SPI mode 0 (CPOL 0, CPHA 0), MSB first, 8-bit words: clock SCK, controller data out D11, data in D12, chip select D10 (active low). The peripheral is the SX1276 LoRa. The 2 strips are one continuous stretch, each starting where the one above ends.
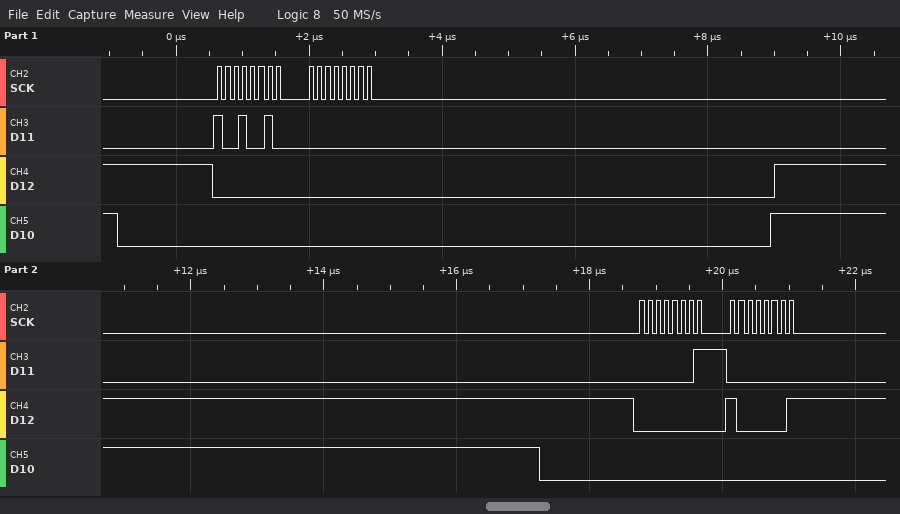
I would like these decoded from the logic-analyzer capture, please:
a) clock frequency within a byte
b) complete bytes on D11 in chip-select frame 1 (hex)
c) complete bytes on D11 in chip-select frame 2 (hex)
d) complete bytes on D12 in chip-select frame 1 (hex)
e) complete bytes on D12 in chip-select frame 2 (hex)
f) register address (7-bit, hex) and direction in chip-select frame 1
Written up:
8 MHz
92 00
01 00
00 00
00 81
0x12 write
